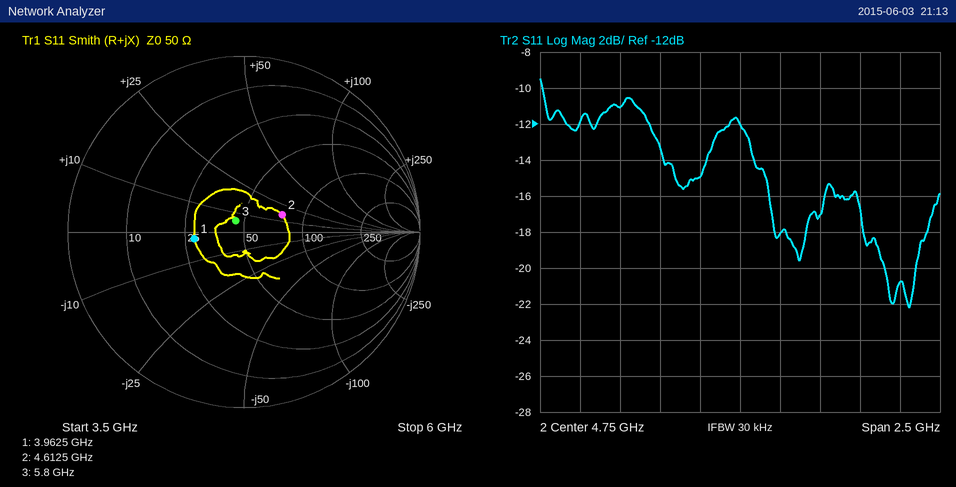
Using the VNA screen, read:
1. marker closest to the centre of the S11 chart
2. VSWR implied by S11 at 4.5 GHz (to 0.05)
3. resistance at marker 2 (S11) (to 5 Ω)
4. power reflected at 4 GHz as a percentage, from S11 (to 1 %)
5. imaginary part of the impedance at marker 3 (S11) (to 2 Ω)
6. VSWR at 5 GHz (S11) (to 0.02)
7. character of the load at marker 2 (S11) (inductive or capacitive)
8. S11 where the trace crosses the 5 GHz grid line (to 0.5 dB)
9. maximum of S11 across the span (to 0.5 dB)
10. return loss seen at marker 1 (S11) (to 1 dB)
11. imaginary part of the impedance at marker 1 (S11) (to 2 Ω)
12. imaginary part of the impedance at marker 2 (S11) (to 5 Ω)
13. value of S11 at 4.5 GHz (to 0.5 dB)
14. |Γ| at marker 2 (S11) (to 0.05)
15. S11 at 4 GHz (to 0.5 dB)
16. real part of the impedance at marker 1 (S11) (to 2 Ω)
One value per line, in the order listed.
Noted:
marker 3
1.45
75 Ω
8 %
+6 Ω
1.28
inductive
-18.0 dB
-9.5 dB
11 dB
-2 Ω
+15 Ω
-15.0 dB
0.25
-11.0 dB
28 Ω
